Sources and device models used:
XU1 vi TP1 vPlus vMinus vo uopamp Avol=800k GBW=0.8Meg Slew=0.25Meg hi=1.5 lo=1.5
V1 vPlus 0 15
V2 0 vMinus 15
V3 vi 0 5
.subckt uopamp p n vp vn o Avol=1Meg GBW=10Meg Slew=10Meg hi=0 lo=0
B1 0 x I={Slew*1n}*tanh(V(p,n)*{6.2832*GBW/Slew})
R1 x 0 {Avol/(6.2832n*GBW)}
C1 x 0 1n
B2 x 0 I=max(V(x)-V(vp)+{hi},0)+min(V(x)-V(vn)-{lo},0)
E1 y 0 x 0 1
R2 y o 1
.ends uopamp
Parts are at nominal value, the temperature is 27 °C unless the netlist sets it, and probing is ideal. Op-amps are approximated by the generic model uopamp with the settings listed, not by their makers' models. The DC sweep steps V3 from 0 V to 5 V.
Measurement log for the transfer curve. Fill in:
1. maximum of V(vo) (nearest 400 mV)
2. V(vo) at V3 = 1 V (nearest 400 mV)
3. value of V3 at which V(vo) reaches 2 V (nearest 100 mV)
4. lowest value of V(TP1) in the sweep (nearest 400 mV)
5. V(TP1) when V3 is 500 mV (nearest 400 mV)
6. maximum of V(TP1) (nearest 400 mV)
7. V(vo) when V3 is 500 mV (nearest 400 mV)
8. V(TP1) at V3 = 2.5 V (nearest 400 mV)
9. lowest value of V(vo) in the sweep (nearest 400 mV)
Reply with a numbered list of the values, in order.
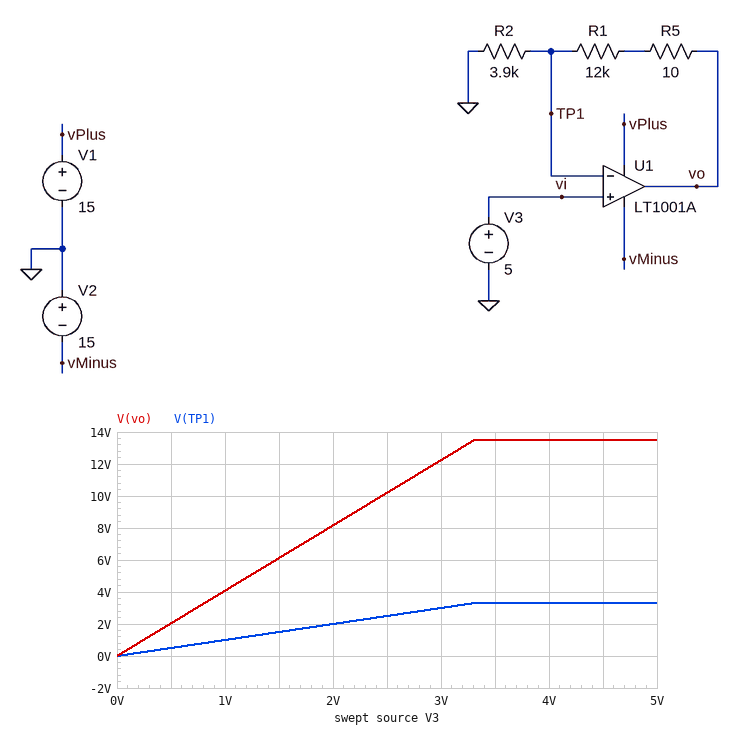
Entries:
1. 13.6 V
2. 4.0 V
3. 500 mV
4. 0 V
5. 400 mV
6. 3.2 V
7. 2.0 V
8. 2.4 V
9. 0 V
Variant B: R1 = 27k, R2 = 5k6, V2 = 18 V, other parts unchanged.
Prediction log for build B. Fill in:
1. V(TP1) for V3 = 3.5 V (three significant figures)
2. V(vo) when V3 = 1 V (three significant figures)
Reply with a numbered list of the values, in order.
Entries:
1. 2.32 V
2. 5.82 V
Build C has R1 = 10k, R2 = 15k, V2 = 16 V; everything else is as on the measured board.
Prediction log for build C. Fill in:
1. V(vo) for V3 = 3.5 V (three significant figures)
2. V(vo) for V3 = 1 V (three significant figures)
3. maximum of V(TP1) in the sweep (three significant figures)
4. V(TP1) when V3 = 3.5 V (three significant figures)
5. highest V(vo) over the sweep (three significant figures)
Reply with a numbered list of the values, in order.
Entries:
1. 5.84 V
2. 1.67 V
3. 5.00 V
4. 3.50 V
5. 8.34 V
